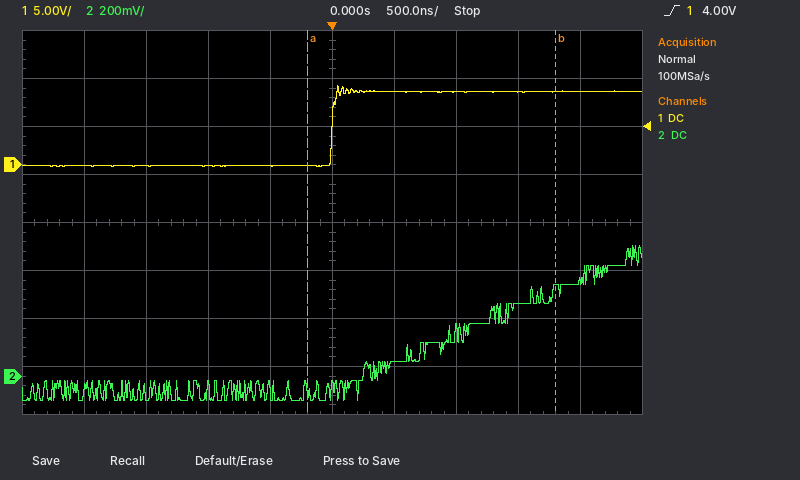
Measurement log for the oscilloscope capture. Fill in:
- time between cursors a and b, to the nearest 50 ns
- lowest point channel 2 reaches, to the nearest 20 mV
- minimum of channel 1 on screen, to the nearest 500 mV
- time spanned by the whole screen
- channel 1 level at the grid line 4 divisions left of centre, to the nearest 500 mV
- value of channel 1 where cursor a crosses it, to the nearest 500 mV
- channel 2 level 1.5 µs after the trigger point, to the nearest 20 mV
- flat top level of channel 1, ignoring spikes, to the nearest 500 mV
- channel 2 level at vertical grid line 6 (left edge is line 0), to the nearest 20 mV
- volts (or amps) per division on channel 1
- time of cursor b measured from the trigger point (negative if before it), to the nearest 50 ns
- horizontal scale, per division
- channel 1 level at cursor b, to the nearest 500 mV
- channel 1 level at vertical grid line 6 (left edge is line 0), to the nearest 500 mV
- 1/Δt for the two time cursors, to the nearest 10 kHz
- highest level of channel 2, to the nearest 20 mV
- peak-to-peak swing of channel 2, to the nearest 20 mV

2.00 µs
-100 mV
0.0 V
5 µs
0.0 V
0.0 V
300 mV
7.5 V
60 mV
5 V
+1.80 µs
500 ns
7.5 V
7.5 V
500 kHz
540 mV
640 mV
